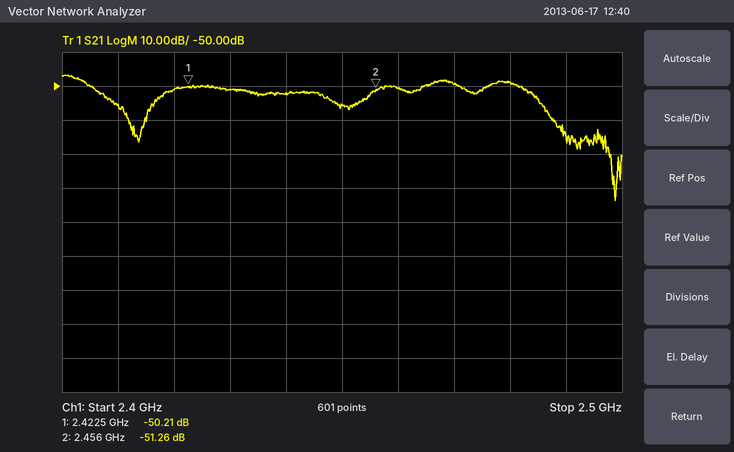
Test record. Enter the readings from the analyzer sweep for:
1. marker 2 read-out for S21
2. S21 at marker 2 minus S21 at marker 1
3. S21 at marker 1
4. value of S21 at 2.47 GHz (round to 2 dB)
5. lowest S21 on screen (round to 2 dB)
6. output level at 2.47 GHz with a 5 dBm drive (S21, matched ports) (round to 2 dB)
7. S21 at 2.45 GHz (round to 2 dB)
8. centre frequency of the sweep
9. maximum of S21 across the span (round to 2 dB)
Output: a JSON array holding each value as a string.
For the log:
["-51.26 dB", "-1.05 dB", "-50.21 dB", "-50 dB", "-84 dB", "-44 dBm", "-56 dB", "2.45 GHz", "-46 dB"]
